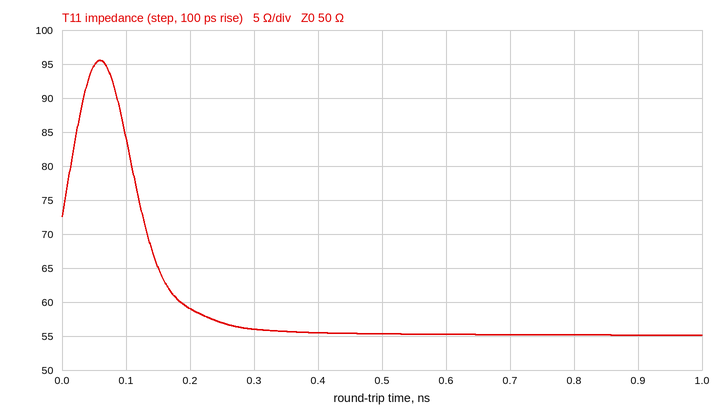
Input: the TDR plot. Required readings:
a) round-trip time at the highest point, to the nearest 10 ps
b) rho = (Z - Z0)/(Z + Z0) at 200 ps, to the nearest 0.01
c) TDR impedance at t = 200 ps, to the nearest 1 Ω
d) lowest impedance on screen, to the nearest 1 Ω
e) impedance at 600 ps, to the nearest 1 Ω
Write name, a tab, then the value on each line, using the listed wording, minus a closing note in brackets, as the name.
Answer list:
round-trip time at the highest point, to the nearest 10 ps	60 ps
rho = (Z - Z0)/(Z + Z0) at 200 ps, to the nearest 0.01	+0.08
TDR impedance at t = 200 ps, to the nearest 1 Ω	59 Ω
lowest impedance on screen, to the nearest 1 Ω	55 Ω
impedance at 600 ps, to the nearest 1 Ω	55 Ω
